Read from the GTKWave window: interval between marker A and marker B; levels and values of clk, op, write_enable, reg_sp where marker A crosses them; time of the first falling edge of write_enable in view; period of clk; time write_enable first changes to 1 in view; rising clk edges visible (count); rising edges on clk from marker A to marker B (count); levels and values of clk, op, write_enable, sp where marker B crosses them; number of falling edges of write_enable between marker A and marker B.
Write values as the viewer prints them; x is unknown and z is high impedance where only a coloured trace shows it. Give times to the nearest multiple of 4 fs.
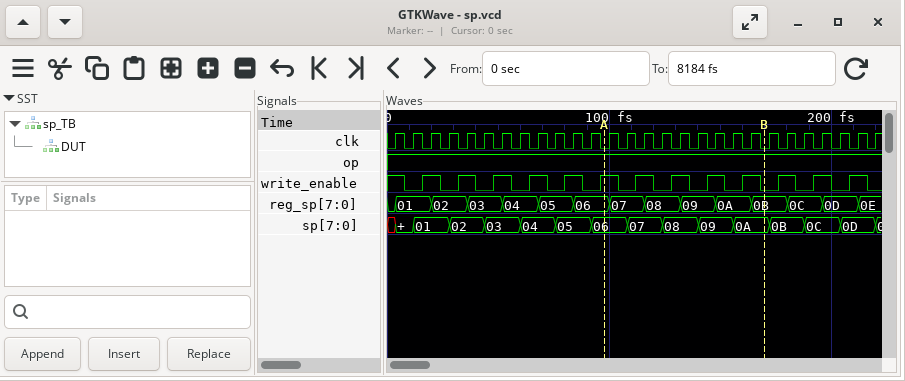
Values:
72 fs
clk=0, op=1, write_enable=1, reg_sp=06
8 fs
8 fs
16 fs
28
9
clk=0, op=1, write_enable=0, sp=0A
5
